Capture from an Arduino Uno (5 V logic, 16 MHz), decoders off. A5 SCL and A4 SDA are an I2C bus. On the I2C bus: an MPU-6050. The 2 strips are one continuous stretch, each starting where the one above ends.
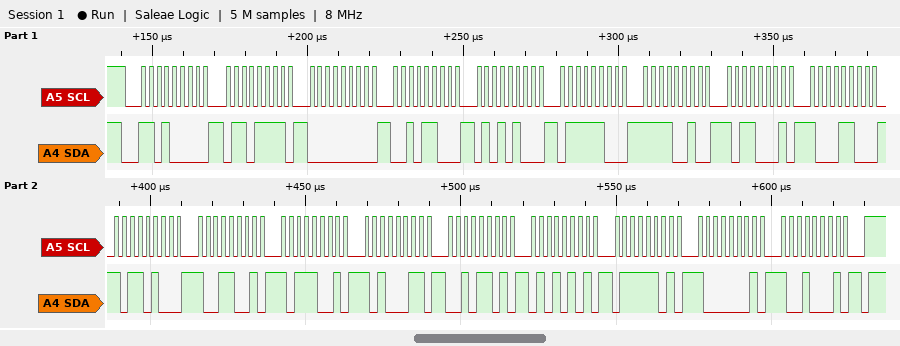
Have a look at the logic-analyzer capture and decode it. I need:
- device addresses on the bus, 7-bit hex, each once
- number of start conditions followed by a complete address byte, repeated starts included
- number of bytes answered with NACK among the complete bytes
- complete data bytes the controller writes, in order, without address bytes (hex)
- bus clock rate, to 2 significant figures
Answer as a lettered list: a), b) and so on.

a) 0x68
b) 1
c) 0
d) 6F 00 2C 54 7C F2 B1 8C B4 99 B9 A3 2D 55 7D 81 91
e) 400 kHz
